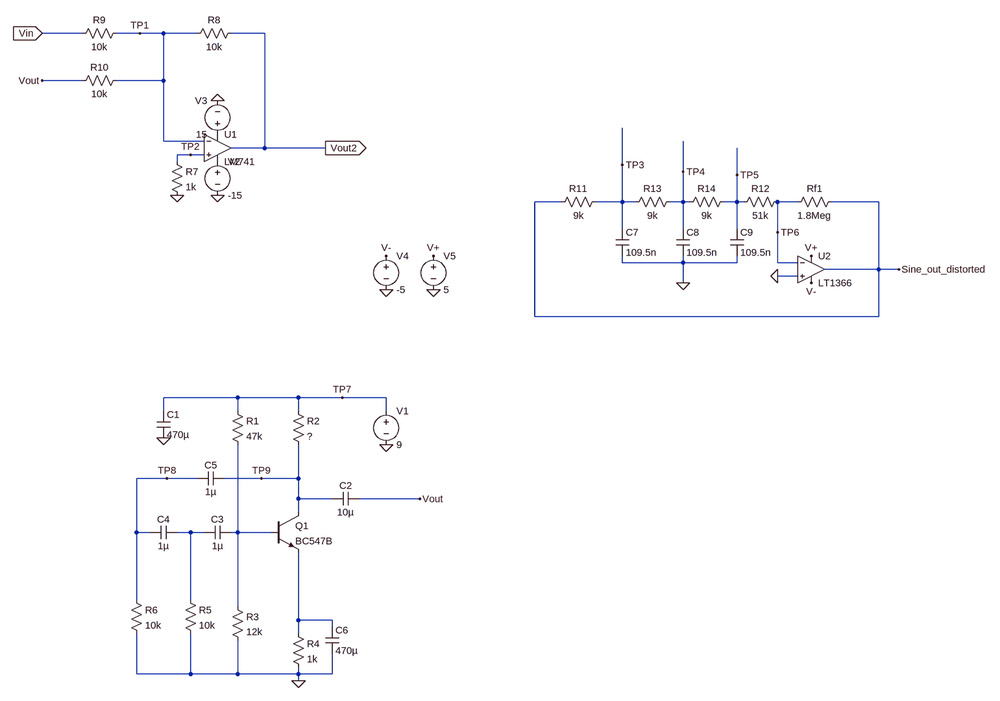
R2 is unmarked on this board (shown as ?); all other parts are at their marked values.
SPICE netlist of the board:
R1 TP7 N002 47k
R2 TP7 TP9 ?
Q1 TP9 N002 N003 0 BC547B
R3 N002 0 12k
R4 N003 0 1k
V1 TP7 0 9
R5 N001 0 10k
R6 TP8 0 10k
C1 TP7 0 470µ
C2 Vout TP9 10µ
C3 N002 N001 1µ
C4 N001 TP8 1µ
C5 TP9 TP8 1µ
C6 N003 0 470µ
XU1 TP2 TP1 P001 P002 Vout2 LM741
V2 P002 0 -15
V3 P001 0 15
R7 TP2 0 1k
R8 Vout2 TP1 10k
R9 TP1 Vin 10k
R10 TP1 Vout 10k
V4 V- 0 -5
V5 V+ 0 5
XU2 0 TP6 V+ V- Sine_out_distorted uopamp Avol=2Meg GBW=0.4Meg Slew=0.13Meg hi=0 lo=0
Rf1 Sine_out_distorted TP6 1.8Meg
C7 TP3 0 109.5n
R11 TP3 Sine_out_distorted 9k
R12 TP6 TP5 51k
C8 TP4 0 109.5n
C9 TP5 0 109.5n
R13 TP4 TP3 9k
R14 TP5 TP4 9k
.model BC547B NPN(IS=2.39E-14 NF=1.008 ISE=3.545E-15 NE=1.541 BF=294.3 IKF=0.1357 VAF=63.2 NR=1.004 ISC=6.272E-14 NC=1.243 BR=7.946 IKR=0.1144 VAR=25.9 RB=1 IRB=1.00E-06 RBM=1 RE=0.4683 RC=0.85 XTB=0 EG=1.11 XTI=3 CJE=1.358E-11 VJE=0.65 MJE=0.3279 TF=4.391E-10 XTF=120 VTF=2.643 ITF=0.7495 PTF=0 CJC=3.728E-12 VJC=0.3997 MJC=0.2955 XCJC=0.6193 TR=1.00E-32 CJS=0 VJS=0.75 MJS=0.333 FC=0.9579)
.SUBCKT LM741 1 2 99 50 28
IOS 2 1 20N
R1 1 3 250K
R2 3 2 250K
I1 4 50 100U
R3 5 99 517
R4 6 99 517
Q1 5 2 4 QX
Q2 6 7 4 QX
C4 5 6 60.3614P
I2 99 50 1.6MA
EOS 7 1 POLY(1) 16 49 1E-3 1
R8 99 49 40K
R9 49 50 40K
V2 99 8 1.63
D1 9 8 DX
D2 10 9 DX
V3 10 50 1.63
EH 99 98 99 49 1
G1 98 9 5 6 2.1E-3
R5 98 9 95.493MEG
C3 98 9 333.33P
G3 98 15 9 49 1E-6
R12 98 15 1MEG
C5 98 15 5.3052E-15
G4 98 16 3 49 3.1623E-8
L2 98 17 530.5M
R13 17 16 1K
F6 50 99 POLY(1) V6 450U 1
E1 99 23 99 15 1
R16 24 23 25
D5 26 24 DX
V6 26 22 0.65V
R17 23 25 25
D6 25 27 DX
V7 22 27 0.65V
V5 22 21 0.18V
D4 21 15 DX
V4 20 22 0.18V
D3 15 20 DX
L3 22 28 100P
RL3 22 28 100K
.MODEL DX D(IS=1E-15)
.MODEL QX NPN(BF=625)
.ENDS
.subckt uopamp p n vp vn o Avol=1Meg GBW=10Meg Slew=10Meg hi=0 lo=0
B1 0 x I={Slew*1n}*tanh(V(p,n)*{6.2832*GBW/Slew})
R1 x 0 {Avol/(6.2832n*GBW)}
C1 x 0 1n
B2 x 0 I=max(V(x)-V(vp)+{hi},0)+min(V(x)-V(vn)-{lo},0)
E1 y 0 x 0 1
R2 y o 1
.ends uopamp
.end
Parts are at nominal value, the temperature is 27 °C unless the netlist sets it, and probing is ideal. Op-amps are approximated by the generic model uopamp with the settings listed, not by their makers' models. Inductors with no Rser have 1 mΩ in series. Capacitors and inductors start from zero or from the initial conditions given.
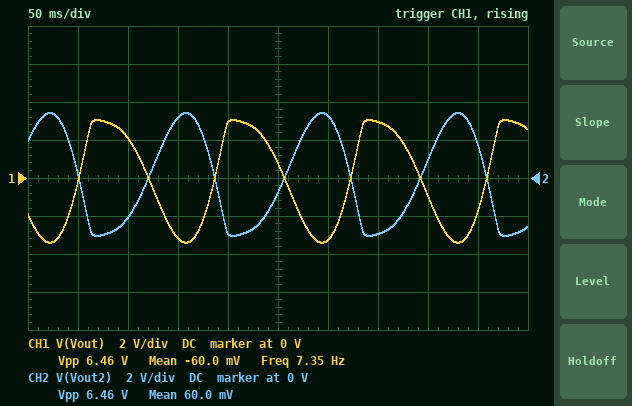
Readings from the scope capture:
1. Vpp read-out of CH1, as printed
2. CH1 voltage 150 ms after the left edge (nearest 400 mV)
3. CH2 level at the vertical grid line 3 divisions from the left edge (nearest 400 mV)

6.46 V
-3.2 V
3.2 V
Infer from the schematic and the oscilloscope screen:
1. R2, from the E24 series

3.3 kΩ
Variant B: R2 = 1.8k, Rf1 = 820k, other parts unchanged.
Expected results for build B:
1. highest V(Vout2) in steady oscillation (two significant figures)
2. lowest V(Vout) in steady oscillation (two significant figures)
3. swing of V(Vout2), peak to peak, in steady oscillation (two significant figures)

2.0 V
-2.0 V
3.8 V
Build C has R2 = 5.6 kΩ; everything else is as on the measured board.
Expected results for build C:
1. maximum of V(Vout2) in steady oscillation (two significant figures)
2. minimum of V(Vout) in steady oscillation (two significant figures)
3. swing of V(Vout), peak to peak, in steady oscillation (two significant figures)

1.8 V
-1.8 V
3.3 V
